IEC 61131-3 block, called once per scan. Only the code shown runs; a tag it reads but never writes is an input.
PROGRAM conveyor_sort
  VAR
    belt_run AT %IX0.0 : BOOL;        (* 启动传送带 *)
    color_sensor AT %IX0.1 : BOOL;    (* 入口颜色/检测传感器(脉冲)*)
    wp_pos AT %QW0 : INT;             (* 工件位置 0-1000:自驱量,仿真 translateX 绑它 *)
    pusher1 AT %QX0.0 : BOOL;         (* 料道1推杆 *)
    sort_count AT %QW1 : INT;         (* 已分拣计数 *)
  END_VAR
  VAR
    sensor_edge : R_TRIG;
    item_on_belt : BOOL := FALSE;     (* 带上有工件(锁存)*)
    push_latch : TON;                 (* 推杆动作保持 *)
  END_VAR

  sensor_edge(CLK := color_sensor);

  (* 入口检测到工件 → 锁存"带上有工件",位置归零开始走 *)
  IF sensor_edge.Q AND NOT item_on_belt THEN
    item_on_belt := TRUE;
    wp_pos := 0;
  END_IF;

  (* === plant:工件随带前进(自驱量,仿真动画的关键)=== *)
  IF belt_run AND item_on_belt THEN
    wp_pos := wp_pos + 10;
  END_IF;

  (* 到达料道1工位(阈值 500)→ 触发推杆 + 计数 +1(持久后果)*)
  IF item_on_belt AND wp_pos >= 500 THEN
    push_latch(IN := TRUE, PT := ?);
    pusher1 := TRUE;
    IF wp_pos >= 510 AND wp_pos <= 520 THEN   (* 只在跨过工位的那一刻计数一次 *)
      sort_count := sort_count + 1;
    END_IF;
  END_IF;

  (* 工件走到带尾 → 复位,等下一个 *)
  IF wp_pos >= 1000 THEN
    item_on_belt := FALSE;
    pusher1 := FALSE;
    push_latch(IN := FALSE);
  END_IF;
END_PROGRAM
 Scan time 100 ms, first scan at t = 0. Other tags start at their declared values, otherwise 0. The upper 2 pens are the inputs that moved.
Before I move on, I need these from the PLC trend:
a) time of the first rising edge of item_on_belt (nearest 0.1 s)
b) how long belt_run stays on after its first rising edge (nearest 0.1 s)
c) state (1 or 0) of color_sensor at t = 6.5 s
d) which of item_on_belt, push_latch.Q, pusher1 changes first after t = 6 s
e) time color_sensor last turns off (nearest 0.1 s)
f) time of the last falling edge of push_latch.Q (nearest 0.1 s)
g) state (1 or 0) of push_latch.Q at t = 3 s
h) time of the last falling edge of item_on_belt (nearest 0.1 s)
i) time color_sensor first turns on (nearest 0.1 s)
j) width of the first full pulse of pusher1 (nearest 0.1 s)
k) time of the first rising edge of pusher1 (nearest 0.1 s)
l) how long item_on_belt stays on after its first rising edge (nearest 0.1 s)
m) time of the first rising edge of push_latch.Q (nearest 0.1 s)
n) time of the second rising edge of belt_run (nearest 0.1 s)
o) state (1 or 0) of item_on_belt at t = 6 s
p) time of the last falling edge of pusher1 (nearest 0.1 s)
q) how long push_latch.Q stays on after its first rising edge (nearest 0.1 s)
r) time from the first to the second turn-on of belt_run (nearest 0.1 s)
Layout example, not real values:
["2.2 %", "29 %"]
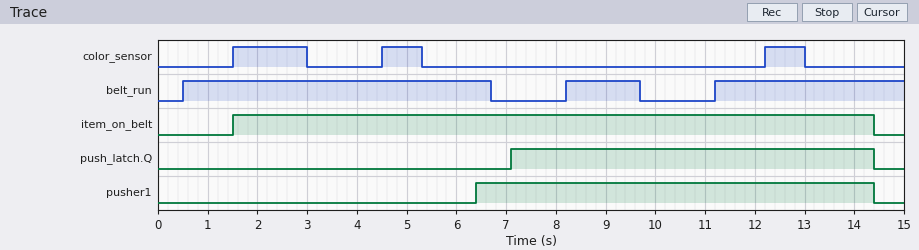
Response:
["1.5 s", "6.2 s", "0", "pusher1", "13.0 s", "14.4 s", "0", "14.4 s", "1.5 s", "8.0 s", "6.4 s", "12.9 s", "7.1 s", "8.2 s", "1", "14.4 s", "7.3 s", "7.7 s"]
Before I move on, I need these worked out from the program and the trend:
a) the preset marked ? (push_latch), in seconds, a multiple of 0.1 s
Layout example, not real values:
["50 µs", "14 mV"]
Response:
["0.7 s"]
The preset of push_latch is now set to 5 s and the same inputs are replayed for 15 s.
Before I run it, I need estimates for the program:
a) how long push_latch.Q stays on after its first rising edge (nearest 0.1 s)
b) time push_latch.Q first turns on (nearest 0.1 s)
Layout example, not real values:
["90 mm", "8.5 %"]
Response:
["3.0 s", "11.4 s"]
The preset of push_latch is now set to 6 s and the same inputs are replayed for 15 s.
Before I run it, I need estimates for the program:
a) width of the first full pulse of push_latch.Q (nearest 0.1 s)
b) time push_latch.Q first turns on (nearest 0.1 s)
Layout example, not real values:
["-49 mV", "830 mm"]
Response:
["2.0 s", "12.4 s"]
